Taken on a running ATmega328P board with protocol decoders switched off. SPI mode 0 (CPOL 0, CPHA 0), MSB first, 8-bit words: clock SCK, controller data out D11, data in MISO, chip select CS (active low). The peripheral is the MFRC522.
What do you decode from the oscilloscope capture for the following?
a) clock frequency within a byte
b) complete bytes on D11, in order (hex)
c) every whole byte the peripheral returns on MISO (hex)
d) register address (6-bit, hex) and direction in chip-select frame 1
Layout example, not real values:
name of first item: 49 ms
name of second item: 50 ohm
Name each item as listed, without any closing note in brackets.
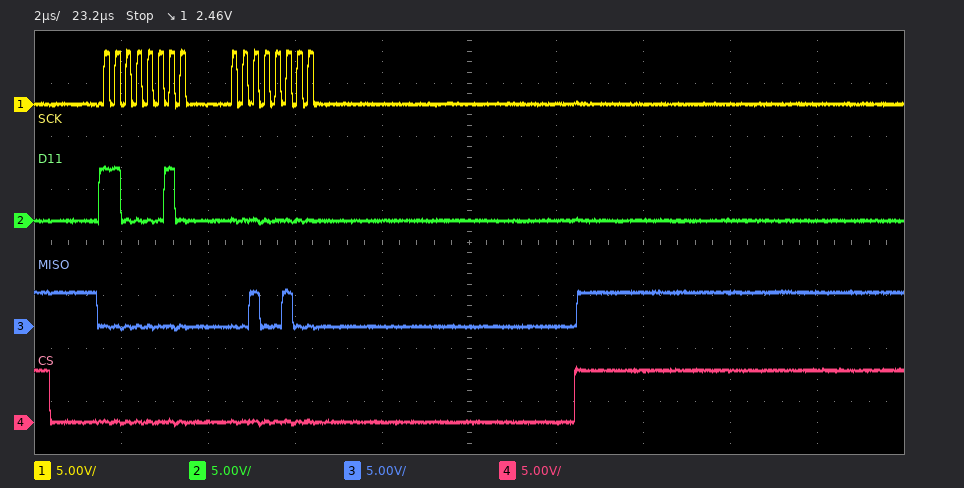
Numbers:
clock frequency within a byte: 4 MHz
complete bytes on D11, in order: 0xC2 0x00
every whole byte the peripheral returns on MISO: 0x00 0x24
register address (6-bit, hex) and direction in chip-select frame 1: 0x21 read
